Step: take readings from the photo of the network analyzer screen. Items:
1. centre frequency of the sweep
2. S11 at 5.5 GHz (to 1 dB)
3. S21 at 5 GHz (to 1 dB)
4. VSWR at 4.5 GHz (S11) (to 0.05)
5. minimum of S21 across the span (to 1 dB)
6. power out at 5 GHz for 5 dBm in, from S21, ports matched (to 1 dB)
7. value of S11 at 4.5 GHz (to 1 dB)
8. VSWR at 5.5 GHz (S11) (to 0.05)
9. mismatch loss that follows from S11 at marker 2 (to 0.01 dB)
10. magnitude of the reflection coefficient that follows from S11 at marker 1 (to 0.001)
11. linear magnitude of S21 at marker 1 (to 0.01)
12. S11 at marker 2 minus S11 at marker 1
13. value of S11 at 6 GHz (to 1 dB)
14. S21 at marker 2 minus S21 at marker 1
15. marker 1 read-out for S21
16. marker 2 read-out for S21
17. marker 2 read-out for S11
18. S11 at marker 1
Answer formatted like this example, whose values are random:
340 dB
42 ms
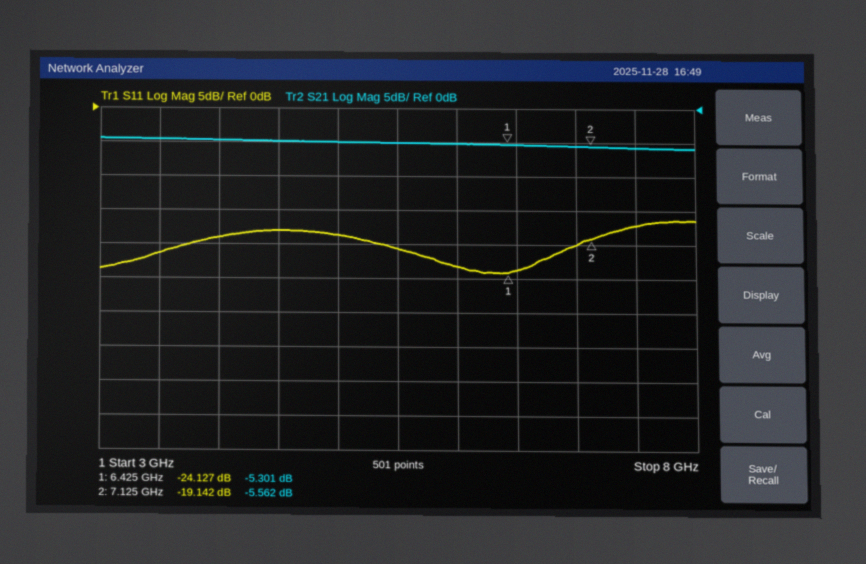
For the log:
5.5 GHz
-21 dB
-5 dB
1.30
-6 dB
0 dBm
-18 dB
1.20
0.05 dB
0.062
0.54
4.985 dB
-23 dB
-0.261 dB
-5.301 dB
-5.562 dB
-19.142 dB
-24.127 dB
